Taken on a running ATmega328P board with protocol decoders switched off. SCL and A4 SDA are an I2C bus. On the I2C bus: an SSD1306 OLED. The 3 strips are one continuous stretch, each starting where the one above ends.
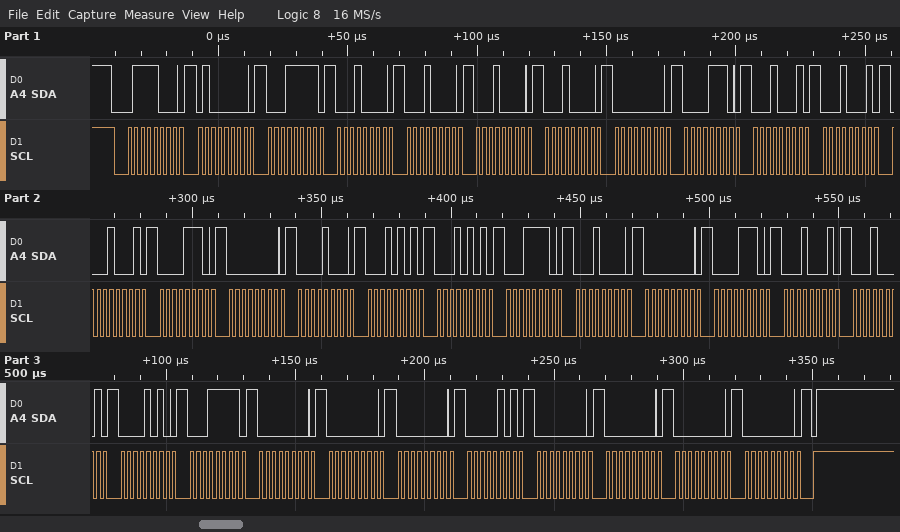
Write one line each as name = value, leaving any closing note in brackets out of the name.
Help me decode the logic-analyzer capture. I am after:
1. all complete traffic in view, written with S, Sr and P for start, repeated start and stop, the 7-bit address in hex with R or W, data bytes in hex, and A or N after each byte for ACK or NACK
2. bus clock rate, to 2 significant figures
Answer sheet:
all complete traffic in view, written with S, Sr and P for start, repeated start and stop, the 7-bit address in hex with R or W, data bytes in hex, and A or N after each byte for ACK or NACK = S 3CW A 40 A 1F A 10 A 10 A 10 A 10 A 00 A 0E A 11 A 11 A 11 A 0E A 00 A 08 A 15 A 15 A 1E A 10 A 00 A 0E A 11 A 11 A 0A A 1F A 00 A 00 A 00 A 05 A 00 A 00 A 00 A 00 A P
bus clock rate, to 2 significant figures = 400 kHz
